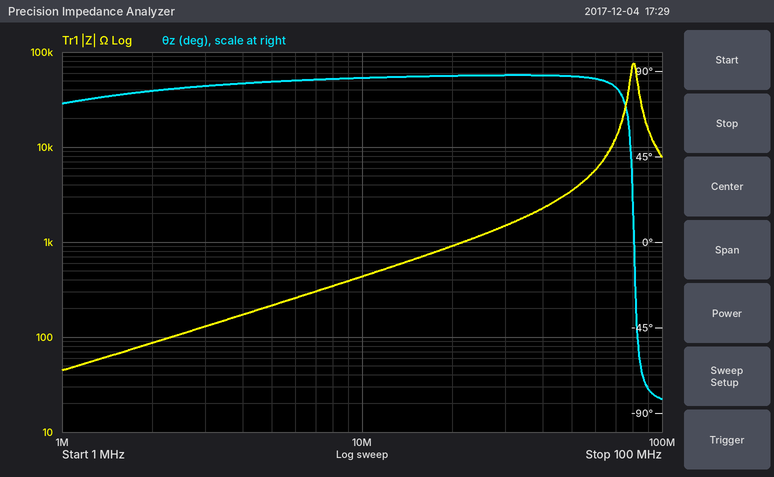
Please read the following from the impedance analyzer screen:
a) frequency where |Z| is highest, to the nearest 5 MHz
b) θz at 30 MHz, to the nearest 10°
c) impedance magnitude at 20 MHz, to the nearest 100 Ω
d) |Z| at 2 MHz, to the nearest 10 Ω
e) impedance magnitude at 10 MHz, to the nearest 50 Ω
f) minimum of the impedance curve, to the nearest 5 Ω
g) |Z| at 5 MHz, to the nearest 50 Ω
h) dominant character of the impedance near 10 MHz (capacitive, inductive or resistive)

80 MHz
90°
900 Ω
90 Ω
450 Ω
45 Ω
200 Ω
inductive
